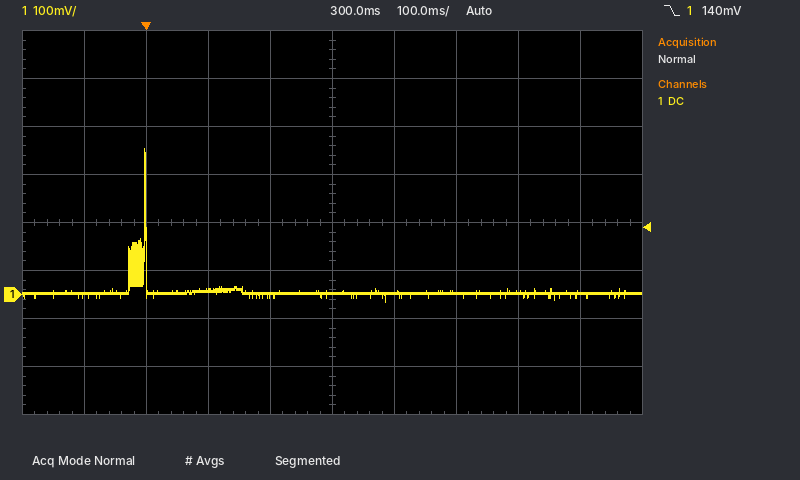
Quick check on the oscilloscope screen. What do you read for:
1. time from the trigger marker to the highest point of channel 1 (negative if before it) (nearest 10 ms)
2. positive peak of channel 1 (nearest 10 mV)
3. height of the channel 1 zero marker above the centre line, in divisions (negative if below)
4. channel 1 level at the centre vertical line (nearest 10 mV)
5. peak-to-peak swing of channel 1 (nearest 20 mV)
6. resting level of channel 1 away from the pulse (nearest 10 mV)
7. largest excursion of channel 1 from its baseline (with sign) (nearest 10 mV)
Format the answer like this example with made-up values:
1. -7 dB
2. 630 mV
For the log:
1. 0 ms
2. 300 mV
3. -1.5 div
4. 0 mV
5. 320 mV
6. 0 mV
7. +300 mV
